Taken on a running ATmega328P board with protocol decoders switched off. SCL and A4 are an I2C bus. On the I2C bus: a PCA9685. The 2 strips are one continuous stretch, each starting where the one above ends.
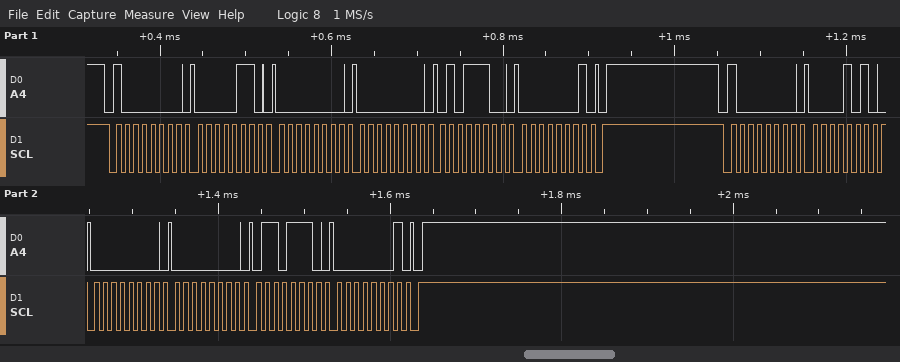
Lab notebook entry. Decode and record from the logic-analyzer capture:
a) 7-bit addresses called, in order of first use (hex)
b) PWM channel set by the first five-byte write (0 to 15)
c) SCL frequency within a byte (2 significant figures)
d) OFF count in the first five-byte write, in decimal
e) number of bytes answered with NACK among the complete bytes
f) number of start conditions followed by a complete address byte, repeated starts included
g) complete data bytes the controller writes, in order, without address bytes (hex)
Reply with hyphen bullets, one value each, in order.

- 0x40
- 0
- 100 kHz
- 348
- 0
- 2
- 06 00 00 5C 01 0A 00 00 6E 01
